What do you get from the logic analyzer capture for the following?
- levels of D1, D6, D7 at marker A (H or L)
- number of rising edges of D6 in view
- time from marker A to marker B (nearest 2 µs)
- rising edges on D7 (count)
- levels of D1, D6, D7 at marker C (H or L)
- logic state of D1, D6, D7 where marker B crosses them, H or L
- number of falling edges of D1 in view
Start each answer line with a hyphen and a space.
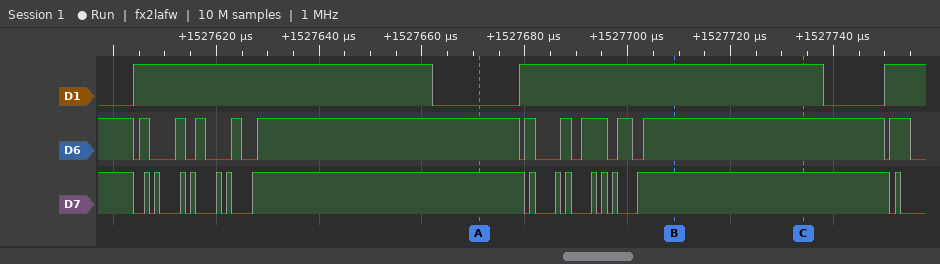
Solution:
- D1=L, D6=H, D7=H
- 11
- 38 µs
- 15
- D1=H, D6=H, D7=H
- D1=H, D6=H, D7=H
- 2
